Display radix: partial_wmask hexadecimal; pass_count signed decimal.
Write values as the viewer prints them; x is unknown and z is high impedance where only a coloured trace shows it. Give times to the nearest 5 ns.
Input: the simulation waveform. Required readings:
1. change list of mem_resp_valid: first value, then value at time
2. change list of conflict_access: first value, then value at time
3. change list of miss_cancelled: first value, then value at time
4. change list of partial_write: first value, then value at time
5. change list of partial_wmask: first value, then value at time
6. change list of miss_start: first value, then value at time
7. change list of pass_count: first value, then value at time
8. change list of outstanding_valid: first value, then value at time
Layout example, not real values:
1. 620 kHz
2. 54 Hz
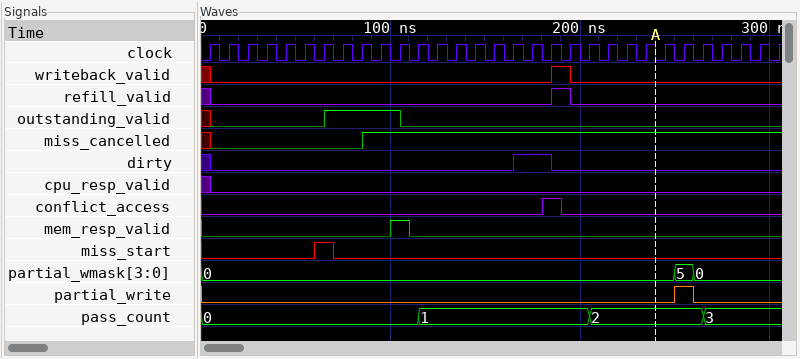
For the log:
1. 0, 1 at 100 ns, 0 at 110 ns
2. 0, 1 at 180 ns, 0 at 190 ns
3. x, 0 at 5 ns, 1 at 85 ns
4. 0, 1 at 250 ns, 0 at 260 ns
5. 0, 5 at 250 ns, 0 at 260 ns
6. 0, 1 at 60 ns, 0 at 70 ns
7. 0, 1 at 115 ns, 2 at 205 ns, 3 at 265 ns
8. x, 0 at 5 ns, 1 at 65 ns, 0 at 105 ns
